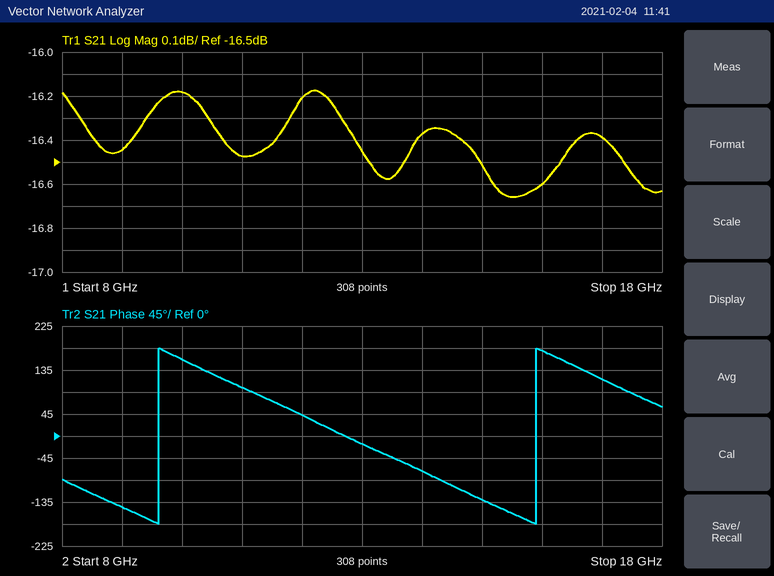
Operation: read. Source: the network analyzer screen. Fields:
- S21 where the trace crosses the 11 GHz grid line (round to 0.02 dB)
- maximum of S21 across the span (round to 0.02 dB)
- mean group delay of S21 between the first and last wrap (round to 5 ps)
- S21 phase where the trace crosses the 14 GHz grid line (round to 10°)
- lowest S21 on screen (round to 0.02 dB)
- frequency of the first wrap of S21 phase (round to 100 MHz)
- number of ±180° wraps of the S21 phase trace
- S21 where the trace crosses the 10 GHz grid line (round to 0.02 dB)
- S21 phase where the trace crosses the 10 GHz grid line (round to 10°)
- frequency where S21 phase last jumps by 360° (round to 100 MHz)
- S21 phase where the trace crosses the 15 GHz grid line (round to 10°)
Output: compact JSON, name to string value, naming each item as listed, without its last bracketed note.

{"S21 where the trace crosses the 11 GHz grid line": "-16.48 dB", "maximum of S21 across the span": "-16.18 dB", "mean group delay of S21 between the first and last wrap": "160 ps", "S21 phase where the trace crosses the 14 GHz grid line": "-70°", "lowest S21 on screen": "-16.66 dB", "frequency of the first wrap of S21 phase": "9.6 GHz", "number of ±180° wraps of the S21 phase trace": "2", "S21 where the trace crosses the 10 GHz grid line": "-16.18 dB", "S21 phase where the trace crosses the 10 GHz grid line": "160°", "frequency where S21 phase last jumps by 360°": "15.9 GHz", "S21 phase where the trace crosses the 15 GHz grid line": "-130°"}
